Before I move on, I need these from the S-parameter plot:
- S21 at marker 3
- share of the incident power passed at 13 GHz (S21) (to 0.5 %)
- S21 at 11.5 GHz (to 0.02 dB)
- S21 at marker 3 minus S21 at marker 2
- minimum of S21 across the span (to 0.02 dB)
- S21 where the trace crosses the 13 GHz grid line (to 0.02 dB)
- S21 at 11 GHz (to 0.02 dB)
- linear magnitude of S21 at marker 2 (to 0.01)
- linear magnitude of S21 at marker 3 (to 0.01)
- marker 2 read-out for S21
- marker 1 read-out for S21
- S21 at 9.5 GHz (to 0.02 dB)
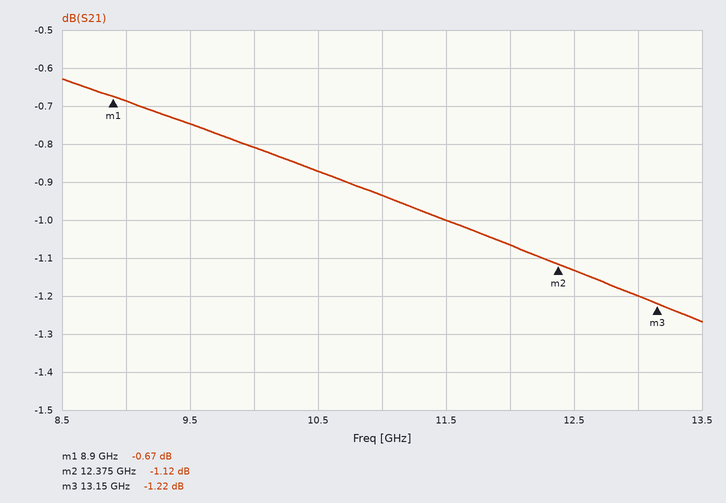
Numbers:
-1.22 dB
76.0 %
-1.00 dB
-0.10 dB
-1.26 dB
-1.20 dB
-0.94 dB
0.88
0.87
-1.12 dB
-0.67 dB
-0.74 dB
